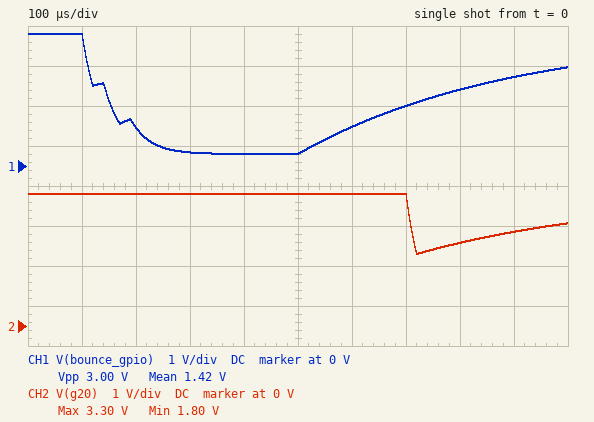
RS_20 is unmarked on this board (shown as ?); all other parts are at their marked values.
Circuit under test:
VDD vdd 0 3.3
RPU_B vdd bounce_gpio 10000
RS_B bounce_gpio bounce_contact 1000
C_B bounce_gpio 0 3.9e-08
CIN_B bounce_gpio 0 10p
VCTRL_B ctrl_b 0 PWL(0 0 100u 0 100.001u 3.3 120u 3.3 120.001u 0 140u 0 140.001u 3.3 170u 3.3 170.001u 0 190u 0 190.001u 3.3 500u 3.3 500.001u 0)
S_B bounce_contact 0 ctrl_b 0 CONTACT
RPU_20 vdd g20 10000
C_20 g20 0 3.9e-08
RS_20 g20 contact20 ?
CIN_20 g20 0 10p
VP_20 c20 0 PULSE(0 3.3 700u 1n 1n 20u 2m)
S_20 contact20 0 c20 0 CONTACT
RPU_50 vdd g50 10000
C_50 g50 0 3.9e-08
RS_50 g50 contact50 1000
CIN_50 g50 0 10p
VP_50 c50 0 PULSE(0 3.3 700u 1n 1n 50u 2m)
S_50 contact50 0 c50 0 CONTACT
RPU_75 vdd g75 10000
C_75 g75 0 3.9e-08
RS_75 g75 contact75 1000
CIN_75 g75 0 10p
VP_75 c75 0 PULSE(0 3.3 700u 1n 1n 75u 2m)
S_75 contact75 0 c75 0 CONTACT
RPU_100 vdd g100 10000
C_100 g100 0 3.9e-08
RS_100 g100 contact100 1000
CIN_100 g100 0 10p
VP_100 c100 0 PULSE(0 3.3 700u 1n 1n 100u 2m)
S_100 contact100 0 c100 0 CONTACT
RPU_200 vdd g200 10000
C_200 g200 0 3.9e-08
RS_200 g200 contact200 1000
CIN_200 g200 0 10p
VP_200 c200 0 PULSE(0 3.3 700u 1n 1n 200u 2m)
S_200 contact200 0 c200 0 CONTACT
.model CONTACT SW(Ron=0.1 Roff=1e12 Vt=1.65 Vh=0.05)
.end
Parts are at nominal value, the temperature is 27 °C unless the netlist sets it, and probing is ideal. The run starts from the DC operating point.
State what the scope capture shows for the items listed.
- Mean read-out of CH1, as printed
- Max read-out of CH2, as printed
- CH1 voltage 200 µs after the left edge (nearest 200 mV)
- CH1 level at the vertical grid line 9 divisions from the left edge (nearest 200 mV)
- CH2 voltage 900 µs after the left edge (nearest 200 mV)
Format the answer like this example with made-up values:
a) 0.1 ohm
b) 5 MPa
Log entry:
a) 1.42 V
b) 3.30 V
c) 1.0 V
d) 2.2 V
e) 2.4 V
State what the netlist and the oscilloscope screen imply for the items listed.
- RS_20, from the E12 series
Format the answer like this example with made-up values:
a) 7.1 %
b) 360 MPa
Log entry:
a) 820 Ω
